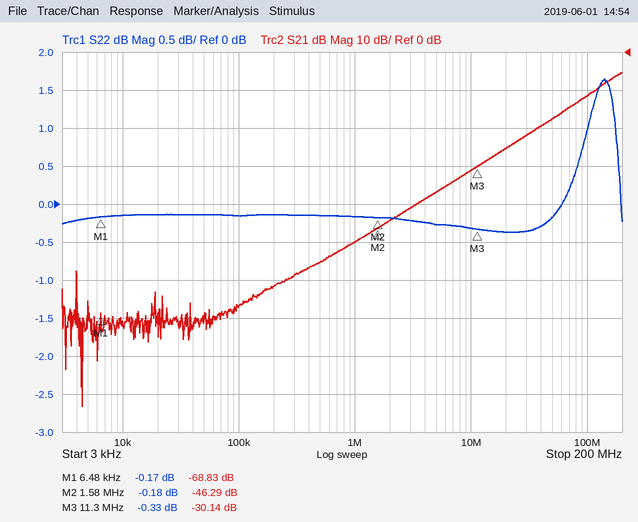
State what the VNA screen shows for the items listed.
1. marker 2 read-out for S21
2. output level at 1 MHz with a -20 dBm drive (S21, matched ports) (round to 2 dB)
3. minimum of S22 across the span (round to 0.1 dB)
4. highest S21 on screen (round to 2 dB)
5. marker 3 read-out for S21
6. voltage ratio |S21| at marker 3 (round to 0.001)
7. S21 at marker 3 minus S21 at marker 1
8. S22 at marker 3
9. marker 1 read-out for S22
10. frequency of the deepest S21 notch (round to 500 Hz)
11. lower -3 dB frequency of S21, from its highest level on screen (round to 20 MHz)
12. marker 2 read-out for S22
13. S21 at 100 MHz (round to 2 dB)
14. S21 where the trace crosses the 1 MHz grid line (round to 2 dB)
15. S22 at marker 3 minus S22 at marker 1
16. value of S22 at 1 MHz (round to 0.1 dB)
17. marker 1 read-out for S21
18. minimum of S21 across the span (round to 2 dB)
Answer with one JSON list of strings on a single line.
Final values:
["-46.29 dB", "-70 dBm", "-0.4 dB", "-6 dB", "-30.14 dB", "0.031", "38.69 dB", "-0.33 dB", "-0.17 dB", "4.5 kHz", "140 MHz", "-0.18 dB", "-12 dB", "-50 dB", "-0.16 dB", "-0.2 dB", "-68.83 dB", "-94 dB"]
